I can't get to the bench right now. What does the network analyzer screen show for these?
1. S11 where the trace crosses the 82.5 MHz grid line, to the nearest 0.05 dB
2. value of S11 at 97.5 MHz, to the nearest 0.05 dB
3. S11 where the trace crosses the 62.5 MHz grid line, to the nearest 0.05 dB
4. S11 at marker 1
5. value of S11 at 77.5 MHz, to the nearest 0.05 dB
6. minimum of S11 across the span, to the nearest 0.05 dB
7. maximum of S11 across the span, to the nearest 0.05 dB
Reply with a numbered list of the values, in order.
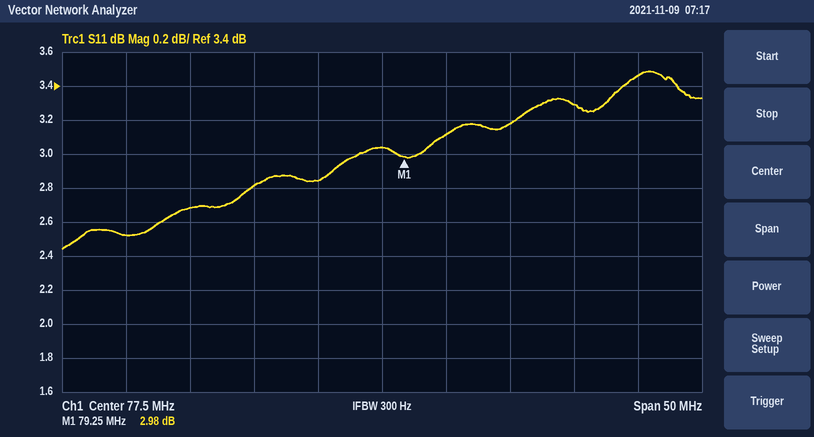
1. 3.10 dB
2. 3.45 dB
3. 2.70 dB
4. 2.98 dB
5. 3.05 dB
6. 2.45 dB
7. 3.50 dB
